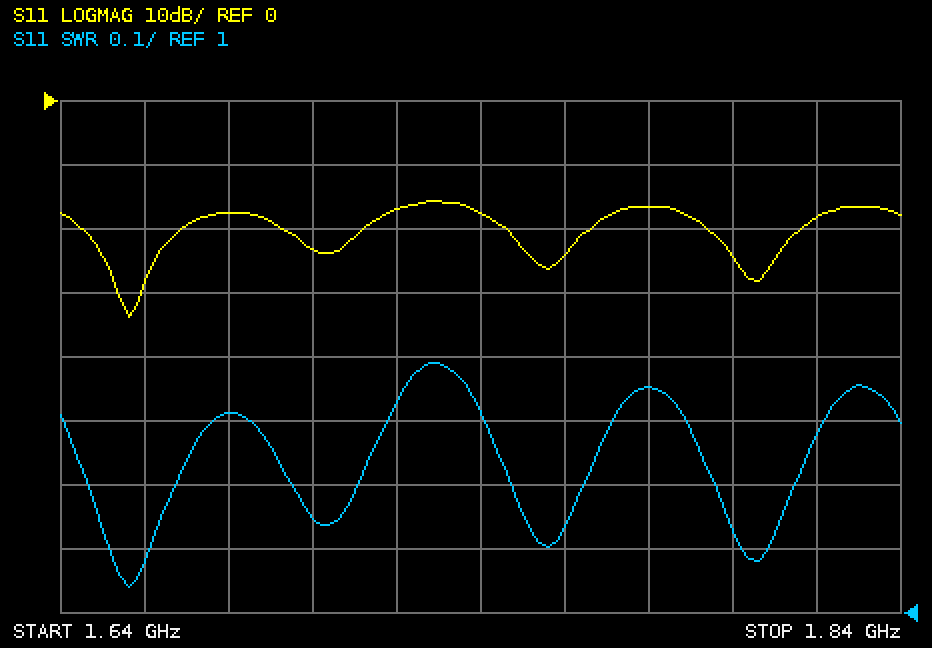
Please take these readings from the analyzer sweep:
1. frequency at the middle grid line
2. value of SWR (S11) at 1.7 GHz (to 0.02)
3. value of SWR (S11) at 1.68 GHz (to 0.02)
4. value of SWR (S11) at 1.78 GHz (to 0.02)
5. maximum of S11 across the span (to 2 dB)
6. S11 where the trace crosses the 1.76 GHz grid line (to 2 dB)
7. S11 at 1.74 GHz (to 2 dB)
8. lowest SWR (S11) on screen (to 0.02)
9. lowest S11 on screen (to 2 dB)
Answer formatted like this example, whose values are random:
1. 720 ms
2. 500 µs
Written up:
1. 1.74 GHz
2. 1.14
3. 1.32
4. 1.36
5. -16 dB
6. -24 dB
7. -18 dB
8. 1.04
9. -34 dB
